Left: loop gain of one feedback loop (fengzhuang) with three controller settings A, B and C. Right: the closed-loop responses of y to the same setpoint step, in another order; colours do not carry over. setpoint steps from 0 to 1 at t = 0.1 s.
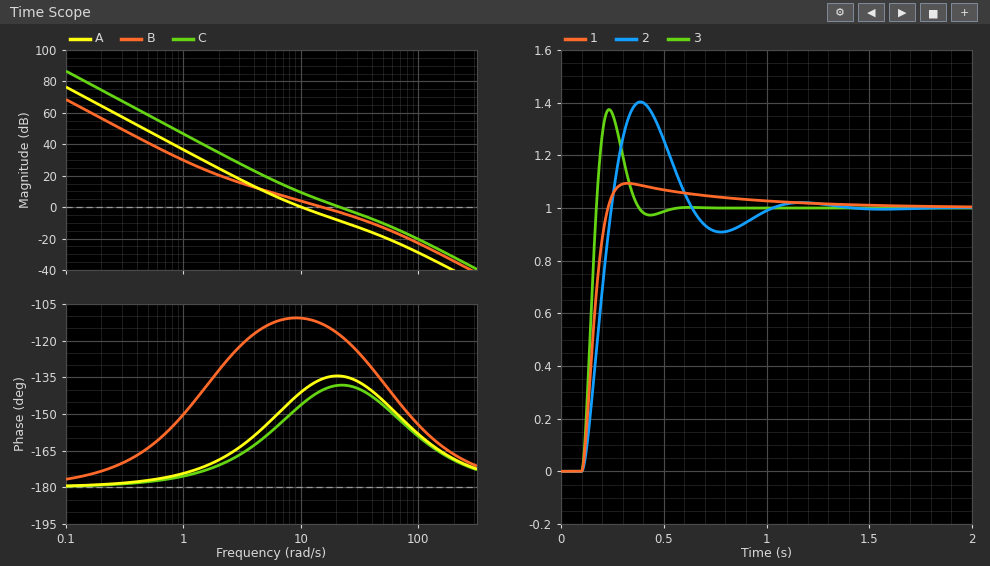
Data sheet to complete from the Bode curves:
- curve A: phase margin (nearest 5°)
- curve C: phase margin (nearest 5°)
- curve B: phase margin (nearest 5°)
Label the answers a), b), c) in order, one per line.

a) 40°
b) 40°
c) 65°
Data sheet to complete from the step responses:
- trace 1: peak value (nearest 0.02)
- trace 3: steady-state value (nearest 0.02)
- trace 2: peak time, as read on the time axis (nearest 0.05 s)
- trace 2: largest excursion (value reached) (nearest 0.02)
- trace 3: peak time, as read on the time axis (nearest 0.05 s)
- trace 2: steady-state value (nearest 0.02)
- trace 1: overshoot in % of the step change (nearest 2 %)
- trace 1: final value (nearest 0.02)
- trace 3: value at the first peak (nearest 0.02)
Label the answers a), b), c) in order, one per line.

a) 1.10
b) 1.00
c) 0.40 s
d) 1.40
e) 0.25 s
f) 1.00
g) 10 %
h) 1.00
i) 1.38
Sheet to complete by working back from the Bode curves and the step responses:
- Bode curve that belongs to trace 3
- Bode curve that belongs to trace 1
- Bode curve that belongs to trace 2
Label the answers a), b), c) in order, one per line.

a) C
b) B
c) A
